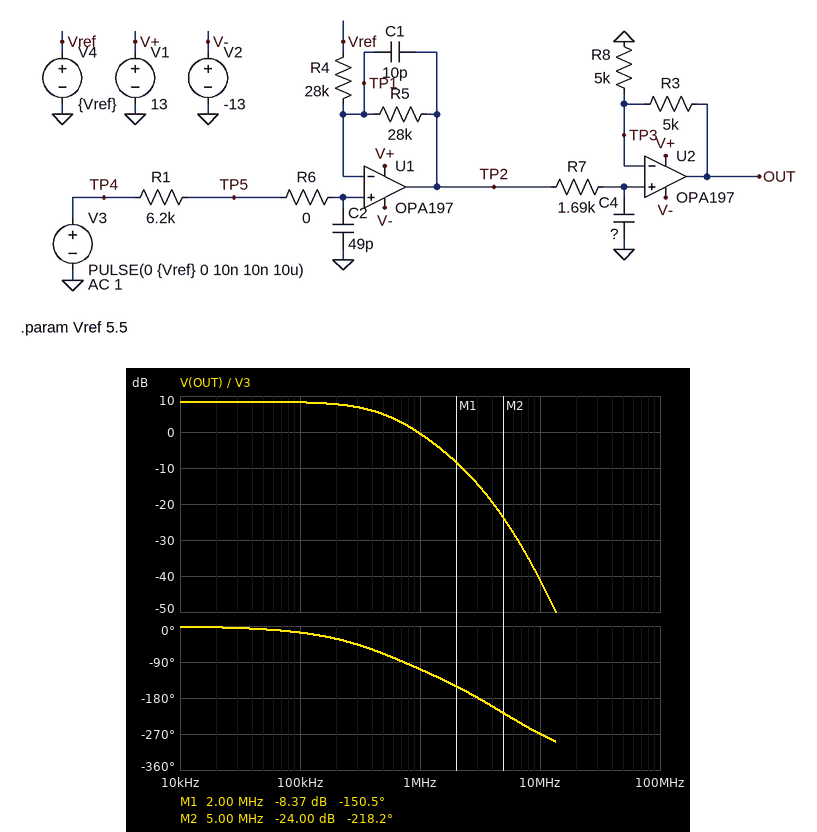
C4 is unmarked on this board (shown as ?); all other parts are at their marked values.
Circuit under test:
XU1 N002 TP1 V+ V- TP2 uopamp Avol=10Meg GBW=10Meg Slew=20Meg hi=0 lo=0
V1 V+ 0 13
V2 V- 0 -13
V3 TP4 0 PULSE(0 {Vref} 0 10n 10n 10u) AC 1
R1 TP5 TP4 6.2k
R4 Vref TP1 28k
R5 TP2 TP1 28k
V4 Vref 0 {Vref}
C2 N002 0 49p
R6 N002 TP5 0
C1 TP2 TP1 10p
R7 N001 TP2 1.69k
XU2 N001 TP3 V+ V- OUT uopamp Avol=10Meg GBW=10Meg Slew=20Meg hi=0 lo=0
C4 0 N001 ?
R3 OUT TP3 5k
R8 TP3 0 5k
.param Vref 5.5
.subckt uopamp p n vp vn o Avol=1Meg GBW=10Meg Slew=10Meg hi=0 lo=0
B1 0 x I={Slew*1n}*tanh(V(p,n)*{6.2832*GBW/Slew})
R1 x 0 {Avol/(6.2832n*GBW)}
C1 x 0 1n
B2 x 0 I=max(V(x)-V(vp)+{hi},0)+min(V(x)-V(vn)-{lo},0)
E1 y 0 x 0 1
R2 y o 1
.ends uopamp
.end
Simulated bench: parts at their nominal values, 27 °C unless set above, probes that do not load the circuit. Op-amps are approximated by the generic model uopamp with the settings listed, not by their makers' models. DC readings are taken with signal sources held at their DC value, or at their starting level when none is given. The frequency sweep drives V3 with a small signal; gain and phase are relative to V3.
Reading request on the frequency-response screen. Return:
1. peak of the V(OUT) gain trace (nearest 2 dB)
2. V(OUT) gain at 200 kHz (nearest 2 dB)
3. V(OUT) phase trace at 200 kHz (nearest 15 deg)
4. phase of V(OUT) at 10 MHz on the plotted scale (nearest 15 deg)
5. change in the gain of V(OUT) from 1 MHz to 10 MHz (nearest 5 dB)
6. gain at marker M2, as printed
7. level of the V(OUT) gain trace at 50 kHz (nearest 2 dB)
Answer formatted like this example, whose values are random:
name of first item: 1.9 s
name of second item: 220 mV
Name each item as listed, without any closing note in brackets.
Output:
peak of the V(OUT) gain trace: 8 dB
V(OUT) gain at 200 kHz: 8 dB
V(OUT) phase trace at 200 kHz: -30 deg
phase of V(OUT) at 10 MHz on the plotted scale: -270 deg
change in the gain of V(OUT) from 1 MHz to 10 MHz: -40 dB
gain at marker M2, as printed: -24.00 dB
level of the V(OUT) gain trace at 50 kHz: 8 dB
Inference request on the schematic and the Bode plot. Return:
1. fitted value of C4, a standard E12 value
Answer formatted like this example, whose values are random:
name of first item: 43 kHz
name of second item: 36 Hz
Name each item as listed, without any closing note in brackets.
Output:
fitted value of C4, a standard E12 value: 33 pF
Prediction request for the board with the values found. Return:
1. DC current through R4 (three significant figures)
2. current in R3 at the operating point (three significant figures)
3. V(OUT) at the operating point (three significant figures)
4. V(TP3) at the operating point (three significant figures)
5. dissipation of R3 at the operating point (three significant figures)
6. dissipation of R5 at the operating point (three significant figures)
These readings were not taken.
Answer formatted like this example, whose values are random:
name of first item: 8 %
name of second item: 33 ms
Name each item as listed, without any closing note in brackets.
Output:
DC current through R4: 196 µA
current in R3 at the operating point: 1.10 mA
V(OUT) at the operating point: -11.0 V
V(TP3) at the operating point: -5.50 V
dissipation of R3 at the operating point: 6.05 mW
dissipation of R5 at the operating point: 1.08 mW
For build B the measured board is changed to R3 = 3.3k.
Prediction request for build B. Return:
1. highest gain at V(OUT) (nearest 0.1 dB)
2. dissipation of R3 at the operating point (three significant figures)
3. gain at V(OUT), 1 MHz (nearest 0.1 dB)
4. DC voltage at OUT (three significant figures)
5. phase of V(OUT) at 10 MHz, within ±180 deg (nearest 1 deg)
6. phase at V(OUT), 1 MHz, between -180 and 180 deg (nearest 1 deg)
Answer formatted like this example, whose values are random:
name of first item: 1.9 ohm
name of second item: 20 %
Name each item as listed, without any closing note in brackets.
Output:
highest gain at V(OUT): 6.8 dB
dissipation of R3 at the operating point: 3.99 mW
gain at V(OUT), 1 MHz: -2.0 dB
DC voltage at OUT: -9.13 V
phase of V(OUT) at 10 MHz, within ±180 deg: 95 deg
phase at V(OUT), 1 MHz, between -180 and 180 deg: -106 deg
